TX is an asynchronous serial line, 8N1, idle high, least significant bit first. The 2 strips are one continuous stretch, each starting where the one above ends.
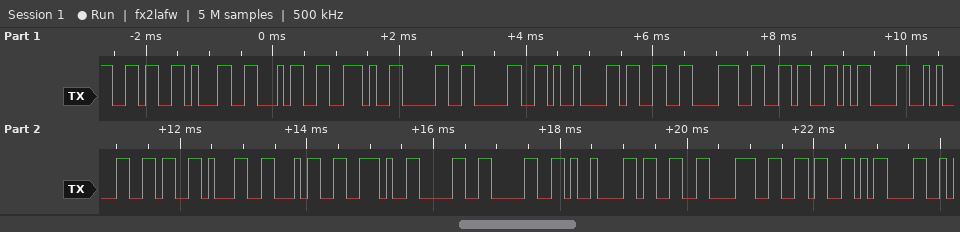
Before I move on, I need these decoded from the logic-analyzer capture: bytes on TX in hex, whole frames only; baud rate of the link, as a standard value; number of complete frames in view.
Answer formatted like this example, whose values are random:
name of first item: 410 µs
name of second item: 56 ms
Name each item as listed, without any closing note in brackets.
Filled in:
bytes on TX in hex, whole frames only: 36 31 34 2E 30 30 09 33 38 36 0D 0A 36 31 34 2E 30 30 09 33 38 36 0D
baud rate of the link, as a standard value: 9600 baud
number of complete frames in view: 23
